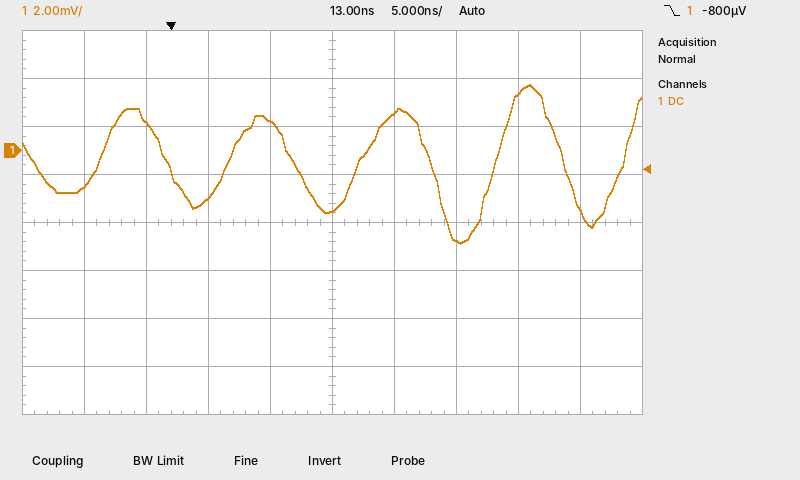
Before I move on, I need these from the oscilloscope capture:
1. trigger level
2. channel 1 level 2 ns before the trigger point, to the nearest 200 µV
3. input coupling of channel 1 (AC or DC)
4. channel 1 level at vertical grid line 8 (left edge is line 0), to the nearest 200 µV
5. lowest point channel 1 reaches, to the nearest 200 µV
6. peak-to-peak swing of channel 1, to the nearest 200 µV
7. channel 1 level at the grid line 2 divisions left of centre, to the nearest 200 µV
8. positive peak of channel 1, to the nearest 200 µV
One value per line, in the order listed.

-800 µV
1.2 mV
DC
2.4 mV
-3.8 mV
6.6 mV
-2.0 mV
2.8 mV
